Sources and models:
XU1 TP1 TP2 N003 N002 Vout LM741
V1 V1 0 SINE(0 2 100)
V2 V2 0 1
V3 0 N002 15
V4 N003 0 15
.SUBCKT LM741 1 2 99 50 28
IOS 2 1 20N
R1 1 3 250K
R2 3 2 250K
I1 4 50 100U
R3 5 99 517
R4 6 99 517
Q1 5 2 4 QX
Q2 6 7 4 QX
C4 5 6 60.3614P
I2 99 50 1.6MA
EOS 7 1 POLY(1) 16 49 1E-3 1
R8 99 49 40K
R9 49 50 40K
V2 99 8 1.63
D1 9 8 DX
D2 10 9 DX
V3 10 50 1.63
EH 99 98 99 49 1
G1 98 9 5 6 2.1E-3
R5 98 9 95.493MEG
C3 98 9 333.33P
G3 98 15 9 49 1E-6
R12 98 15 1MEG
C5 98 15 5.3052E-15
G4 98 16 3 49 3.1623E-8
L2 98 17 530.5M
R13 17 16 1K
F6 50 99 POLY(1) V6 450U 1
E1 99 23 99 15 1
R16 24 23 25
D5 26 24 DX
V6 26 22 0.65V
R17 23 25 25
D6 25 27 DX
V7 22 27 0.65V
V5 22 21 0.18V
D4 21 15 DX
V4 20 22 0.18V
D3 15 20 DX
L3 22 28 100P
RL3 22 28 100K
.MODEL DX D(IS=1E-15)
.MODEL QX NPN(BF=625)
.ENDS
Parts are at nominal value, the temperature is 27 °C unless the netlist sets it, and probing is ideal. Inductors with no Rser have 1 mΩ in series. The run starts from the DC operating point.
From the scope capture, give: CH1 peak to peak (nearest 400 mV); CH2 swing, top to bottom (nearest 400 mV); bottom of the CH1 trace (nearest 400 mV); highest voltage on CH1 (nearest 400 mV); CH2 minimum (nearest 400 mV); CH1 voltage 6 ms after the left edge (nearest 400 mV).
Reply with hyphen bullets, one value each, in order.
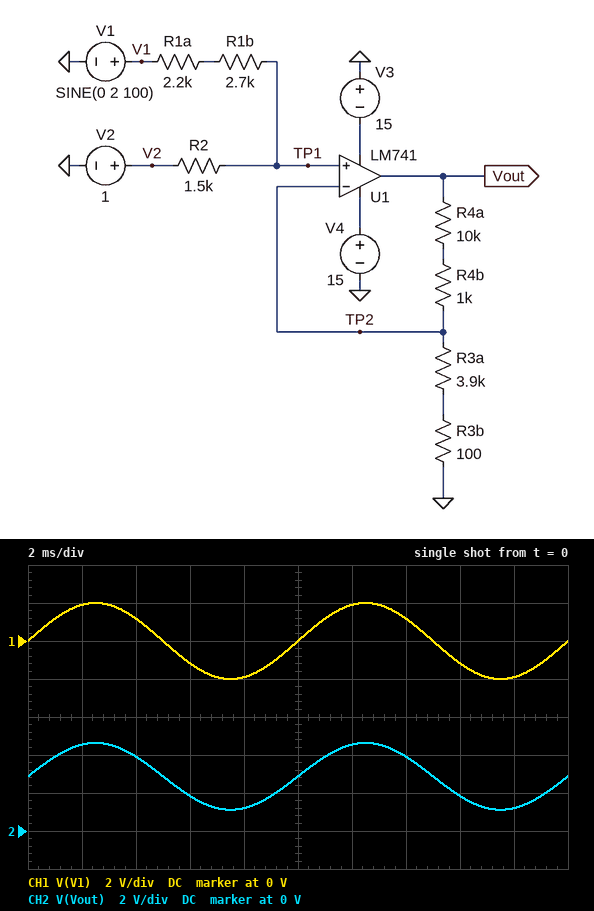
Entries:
- 4.0 V
- 3.6 V
- -2.0 V
- 2.0 V
- 1.2 V
- -1.2 V
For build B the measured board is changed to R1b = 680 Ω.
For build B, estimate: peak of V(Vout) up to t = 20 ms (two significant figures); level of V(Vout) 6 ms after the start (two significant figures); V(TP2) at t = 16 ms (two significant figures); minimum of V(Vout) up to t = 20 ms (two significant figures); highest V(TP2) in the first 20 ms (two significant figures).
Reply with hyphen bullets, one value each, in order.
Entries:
- 5.0 V
- 960 mV
- 260 mV
- -98 mV
- 1.3 V
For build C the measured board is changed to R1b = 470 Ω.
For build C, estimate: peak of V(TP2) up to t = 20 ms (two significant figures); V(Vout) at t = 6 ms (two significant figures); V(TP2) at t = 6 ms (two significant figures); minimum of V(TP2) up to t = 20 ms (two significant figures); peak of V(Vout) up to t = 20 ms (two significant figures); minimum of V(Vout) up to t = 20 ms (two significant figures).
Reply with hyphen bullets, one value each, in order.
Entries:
- 1.4 V
- 820 mV
- 220 mV
- -78 mV
- 5.1 V
- -290 mV
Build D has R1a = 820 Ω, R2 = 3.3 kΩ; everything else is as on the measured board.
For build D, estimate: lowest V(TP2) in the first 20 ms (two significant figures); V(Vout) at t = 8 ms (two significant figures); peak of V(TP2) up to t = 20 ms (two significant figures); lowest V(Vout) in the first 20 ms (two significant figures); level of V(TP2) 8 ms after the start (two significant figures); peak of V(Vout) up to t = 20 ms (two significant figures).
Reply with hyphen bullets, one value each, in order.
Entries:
- -450 mV
- -1.5 V
- 1.5 V
- -1.7 V
- -400 mV
- 5.6 V
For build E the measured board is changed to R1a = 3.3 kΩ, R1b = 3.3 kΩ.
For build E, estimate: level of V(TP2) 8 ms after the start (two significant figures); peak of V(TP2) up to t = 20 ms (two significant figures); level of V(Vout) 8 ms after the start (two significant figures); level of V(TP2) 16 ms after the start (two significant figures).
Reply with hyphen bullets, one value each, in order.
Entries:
- 460 mV
- 1.2 V
- 1.7 V
- 600 mV
